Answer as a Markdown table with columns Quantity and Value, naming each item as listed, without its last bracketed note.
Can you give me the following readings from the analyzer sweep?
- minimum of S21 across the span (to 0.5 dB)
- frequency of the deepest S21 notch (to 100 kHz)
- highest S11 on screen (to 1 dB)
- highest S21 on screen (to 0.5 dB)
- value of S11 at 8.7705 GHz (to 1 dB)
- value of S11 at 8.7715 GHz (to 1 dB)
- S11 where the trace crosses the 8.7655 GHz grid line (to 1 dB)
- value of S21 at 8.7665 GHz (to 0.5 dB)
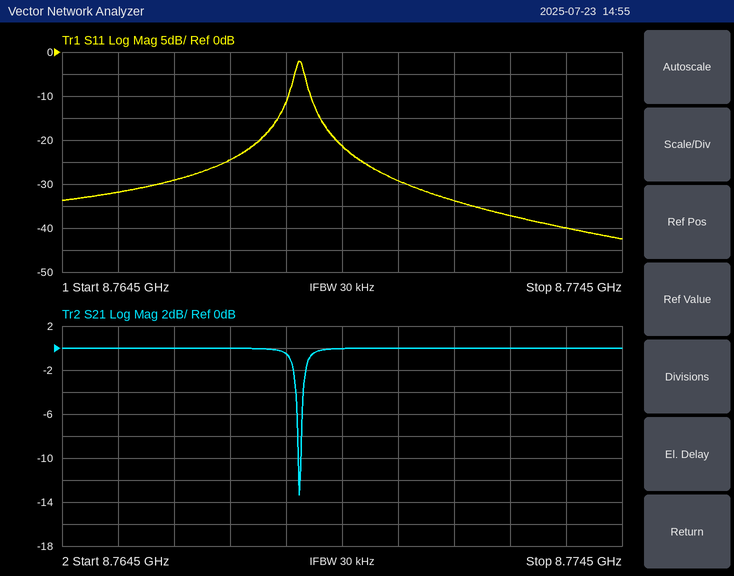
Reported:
| Quantity | Value |
|---|---|
| minimum of S21 across the span | -13.5 dB |
| frequency of the deepest S21 notch | 8.7687 GHz |
| highest S11 on screen | -2 dB |
| highest S21 on screen | 0.0 dB |
| value of S11 at 8.7705 GHz | -29 dB |
| value of S11 at 8.7715 GHz | -34 dB |
| S11 where the trace crosses the 8.7655 GHz grid line | -32 dB |
| value of S21 at 8.7665 GHz | 0.0 dB |
